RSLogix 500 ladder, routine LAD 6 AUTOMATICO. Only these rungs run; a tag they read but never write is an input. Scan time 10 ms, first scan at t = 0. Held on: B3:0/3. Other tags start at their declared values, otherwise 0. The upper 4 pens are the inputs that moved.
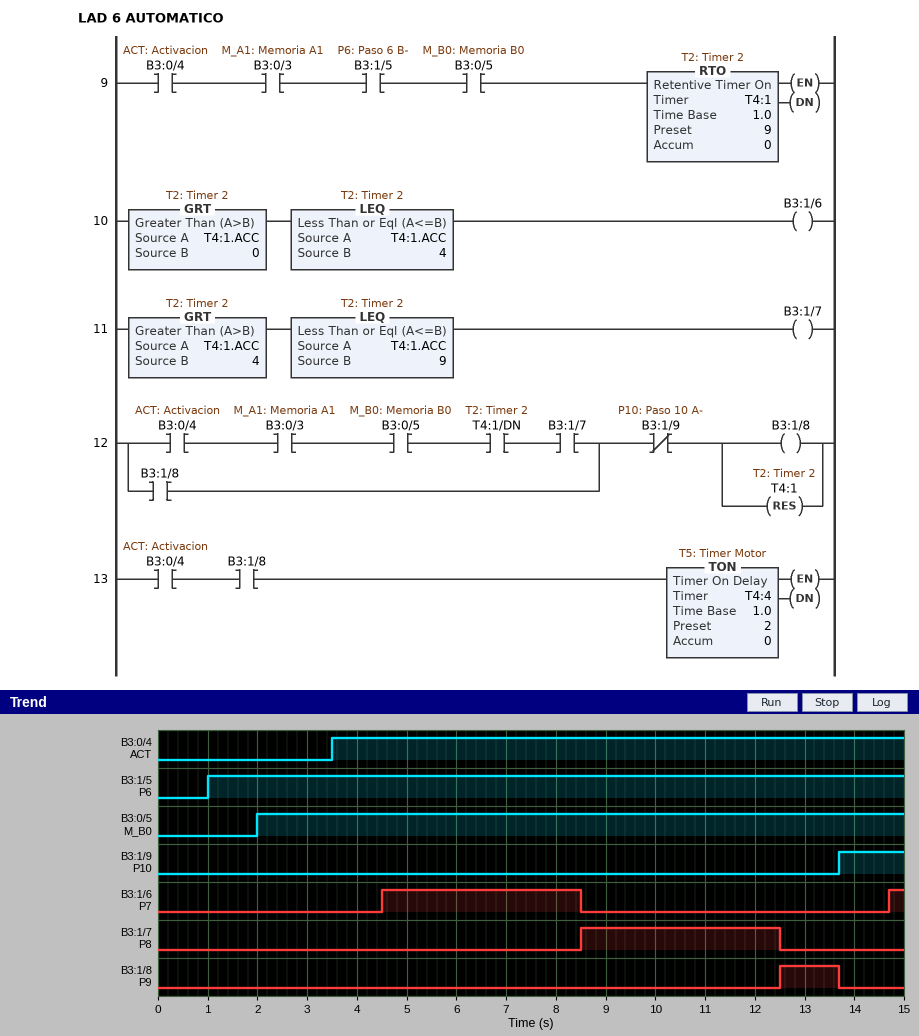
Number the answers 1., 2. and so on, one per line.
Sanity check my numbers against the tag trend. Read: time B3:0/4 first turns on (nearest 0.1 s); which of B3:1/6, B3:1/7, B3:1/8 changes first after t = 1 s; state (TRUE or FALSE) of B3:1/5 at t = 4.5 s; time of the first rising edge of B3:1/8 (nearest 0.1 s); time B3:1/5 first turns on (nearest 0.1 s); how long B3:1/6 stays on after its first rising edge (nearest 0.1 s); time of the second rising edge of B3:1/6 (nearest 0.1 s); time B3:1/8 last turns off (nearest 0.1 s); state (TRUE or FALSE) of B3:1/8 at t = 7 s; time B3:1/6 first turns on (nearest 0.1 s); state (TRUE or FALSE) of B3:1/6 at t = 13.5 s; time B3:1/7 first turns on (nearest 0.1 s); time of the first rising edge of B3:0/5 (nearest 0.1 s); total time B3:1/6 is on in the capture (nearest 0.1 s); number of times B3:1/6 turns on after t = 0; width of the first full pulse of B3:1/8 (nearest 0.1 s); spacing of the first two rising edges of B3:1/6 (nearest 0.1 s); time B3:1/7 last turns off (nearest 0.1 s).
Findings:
1. 3.5 s
2. B3:1/6
3. TRUE
4. 12.5 s
5. 1.0 s
6. 4.0 s
7. 14.7 s
8. 13.7 s
9. FALSE
10. 4.5 s
11. FALSE
12. 8.5 s
13. 2.0 s
14. 4.3 s
15. 2
16. 1.2 s
17. 10.2 s
18. 12.5 s
